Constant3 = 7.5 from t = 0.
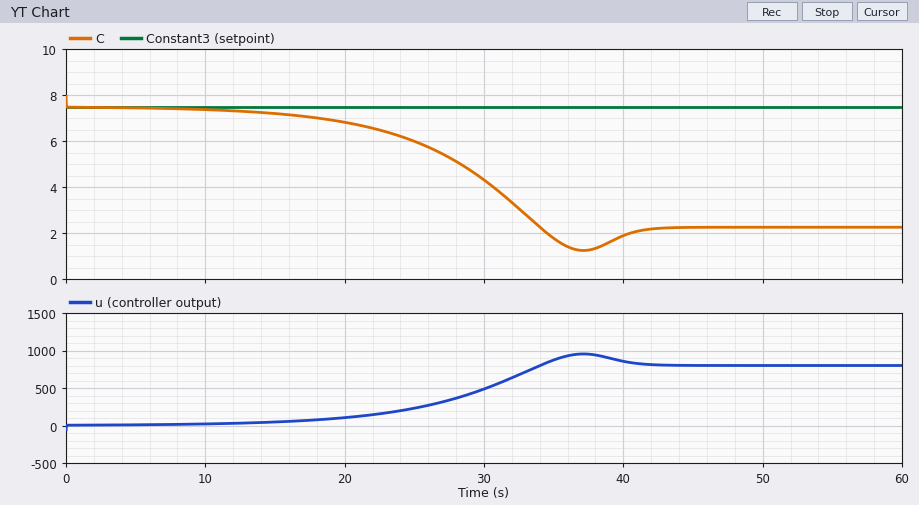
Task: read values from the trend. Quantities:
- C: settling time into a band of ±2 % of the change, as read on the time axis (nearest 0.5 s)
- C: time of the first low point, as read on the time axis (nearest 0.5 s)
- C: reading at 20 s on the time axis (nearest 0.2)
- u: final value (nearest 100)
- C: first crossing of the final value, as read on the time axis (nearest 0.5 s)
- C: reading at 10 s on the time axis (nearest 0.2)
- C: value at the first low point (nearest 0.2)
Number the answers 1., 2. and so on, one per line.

1. 41.5 s
2. 37.0 s
3. 6.8
4. 800
5. 34.0 s
6. 7.4
7. 1.2
